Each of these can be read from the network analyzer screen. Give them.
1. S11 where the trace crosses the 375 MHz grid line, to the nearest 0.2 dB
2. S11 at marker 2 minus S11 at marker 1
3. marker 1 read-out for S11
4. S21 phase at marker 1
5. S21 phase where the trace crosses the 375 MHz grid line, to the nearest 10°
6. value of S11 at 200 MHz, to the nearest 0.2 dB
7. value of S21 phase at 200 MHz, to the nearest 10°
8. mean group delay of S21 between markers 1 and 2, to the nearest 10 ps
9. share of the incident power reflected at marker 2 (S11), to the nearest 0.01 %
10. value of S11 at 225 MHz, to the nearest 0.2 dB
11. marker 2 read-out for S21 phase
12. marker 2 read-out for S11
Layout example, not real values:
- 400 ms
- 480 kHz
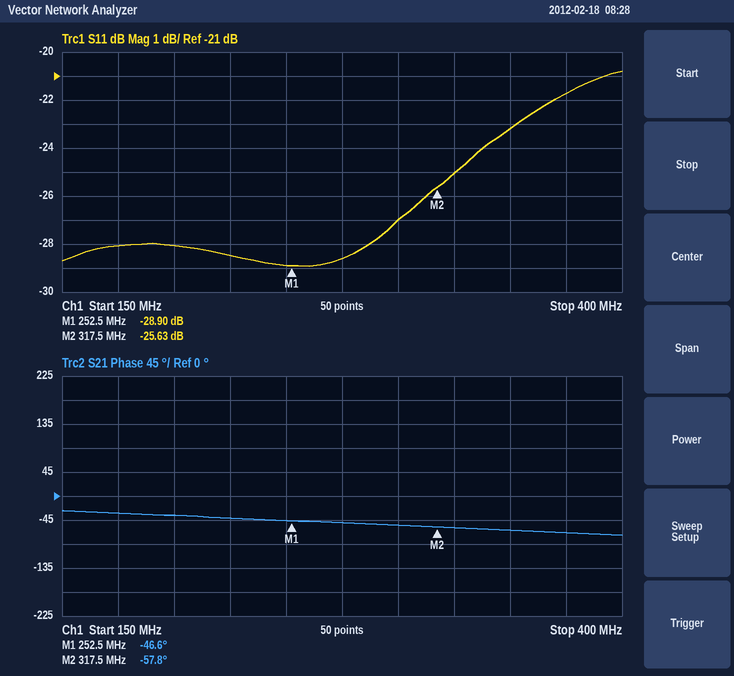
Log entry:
- -21.8 dB
- 3.27 dB
- -28.90 dB
- -46.6°
- -70°
- -28.0 dB
- -40°
- 480 ps
- 0.27 %
- -28.4 dB
- -57.8°
- -25.63 dB
